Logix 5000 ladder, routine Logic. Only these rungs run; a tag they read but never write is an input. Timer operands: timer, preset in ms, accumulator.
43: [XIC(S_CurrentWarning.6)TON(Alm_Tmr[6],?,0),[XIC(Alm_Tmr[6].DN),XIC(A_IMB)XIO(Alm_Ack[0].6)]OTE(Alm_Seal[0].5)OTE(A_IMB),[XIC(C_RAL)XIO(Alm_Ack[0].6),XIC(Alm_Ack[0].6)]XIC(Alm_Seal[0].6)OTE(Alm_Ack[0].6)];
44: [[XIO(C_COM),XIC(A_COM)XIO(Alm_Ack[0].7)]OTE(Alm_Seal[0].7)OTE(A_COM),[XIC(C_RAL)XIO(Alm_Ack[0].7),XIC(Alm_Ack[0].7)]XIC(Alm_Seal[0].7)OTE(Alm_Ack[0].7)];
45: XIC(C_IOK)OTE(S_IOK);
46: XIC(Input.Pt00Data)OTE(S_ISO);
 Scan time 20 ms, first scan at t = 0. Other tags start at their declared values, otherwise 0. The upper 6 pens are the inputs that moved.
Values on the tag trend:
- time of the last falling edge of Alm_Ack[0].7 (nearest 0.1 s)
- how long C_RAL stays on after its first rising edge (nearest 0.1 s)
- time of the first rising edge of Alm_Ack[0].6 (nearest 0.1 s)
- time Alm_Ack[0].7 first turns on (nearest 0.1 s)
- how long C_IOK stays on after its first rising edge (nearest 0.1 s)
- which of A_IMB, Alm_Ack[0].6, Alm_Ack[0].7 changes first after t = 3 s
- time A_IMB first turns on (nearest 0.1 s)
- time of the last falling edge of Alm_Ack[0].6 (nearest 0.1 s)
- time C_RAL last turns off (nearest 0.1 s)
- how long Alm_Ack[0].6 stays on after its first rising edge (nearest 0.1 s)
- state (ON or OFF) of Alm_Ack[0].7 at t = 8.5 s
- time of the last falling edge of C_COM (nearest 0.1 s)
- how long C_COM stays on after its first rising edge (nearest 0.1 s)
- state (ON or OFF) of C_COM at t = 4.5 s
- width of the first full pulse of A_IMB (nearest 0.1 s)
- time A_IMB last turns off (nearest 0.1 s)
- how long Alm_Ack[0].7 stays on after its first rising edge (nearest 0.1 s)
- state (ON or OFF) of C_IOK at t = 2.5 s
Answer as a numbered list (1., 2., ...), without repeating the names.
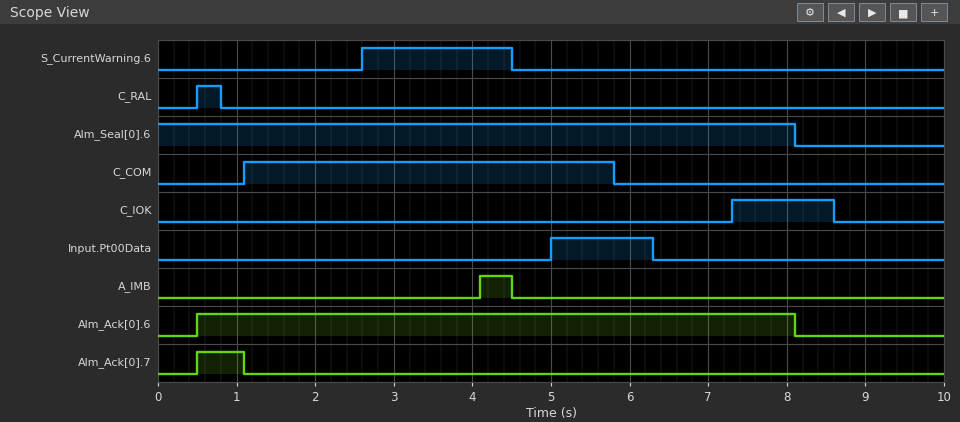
1. 1.1 s
2. 0.3 s
3. 0.5 s
4. 0.5 s
5. 1.3 s
6. A_IMB
7. 4.1 s
8. 8.1 s
9. 0.8 s
10. 7.6 s
11. OFF
12. 5.8 s
13. 4.7 s
14. ON
15. 0.4 s
16. 4.5 s
17. 0.6 s
18. OFF
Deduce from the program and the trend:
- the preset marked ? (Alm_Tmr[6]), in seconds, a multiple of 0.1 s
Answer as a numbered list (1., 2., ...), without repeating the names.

1. 1.5 s
